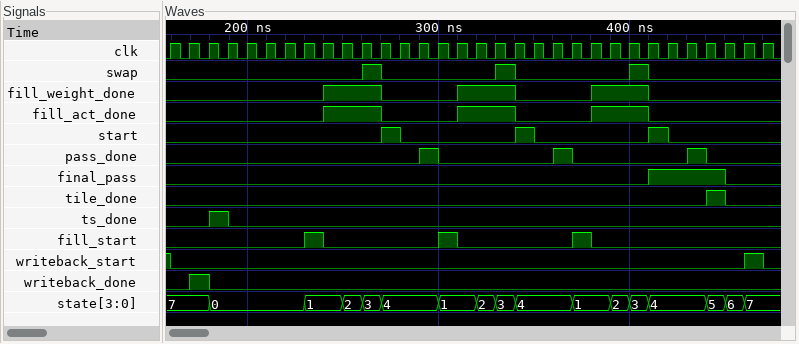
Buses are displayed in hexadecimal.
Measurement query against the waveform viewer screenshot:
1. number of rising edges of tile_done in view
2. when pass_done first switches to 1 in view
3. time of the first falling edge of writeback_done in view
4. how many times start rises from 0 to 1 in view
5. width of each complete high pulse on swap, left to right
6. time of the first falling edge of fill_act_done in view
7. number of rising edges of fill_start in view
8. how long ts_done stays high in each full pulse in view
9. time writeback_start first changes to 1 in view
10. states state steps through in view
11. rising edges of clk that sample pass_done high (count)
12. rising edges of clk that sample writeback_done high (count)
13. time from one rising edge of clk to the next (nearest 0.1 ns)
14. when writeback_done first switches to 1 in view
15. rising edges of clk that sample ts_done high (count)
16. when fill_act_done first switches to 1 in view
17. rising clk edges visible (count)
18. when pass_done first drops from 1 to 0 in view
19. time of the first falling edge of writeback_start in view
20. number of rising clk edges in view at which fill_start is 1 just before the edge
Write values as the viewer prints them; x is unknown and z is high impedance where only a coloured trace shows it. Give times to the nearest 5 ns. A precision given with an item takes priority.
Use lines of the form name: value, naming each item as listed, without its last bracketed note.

number of rising edges of tile_done in view: 1
when pass_done first switches to 1 in view: 290 ns
time of the first falling edge of writeback_done in view: 180 ns
how many times start rises from 0 to 1 in view: 3
width of each complete high pulse on swap, left to right: 10 ns, 10 ns, 10 ns
time of the first falling edge of fill_act_done in view: 270 ns
number of rising edges of fill_start in view: 3
how long ts_done stays high in each full pulse in view: 10 ns
time writeback_start first changes to 1 in view: 460 ns
states state steps through in view: 7, 0, 1, 2, 3, 4, 1, 2, 3, 4, 1, 2, 3, 4, 5, 6, 7
rising edges of clk that sample pass_done high: 3
rising edges of clk that sample writeback_done high: 1
time from one rising edge of clk to the next: 10 ns
when writeback_done first switches to 1 in view: 170 ns
rising edges of clk that sample ts_done high: 1
when fill_act_done first switches to 1 in view: 240 ns
rising clk edges visible: 32
when pass_done first drops from 1 to 0 in view: 300 ns
time of the first falling edge of writeback_start in view: 160 ns
number of rising clk edges in view at which fill_start is 1 just before the edge: 3
